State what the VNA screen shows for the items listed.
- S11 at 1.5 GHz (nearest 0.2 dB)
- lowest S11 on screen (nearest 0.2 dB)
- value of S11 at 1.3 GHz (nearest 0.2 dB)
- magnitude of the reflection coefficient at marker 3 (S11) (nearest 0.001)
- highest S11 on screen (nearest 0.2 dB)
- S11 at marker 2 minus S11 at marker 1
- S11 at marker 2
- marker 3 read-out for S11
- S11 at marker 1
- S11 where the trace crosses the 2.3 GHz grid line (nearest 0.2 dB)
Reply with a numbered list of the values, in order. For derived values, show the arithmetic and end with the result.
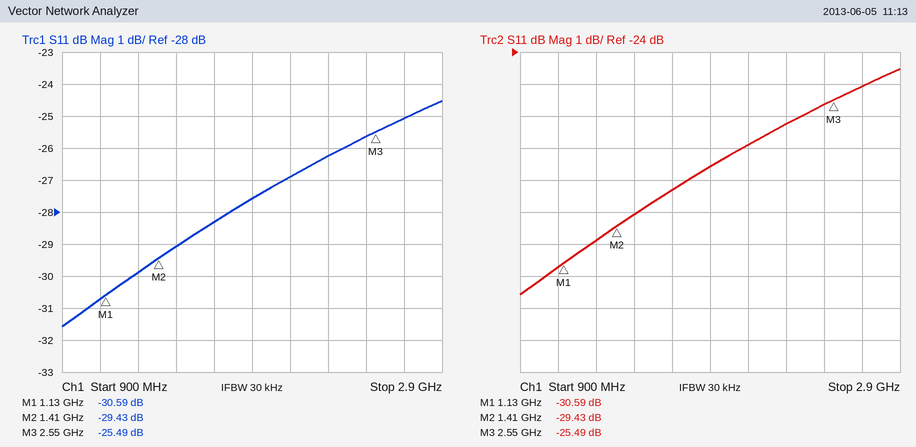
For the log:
1. -29.0 dB
2. -31.6 dB
3. -29.8 dB
4. 10^(-25.49/20) ≈ 0.053
5. -24.6 dB
6. -29.43 − (-30.59) = 1.16 dB
7. -29.43 dB
8. -25.49 dB
9. -30.59 dB
10. -26.2 dB
